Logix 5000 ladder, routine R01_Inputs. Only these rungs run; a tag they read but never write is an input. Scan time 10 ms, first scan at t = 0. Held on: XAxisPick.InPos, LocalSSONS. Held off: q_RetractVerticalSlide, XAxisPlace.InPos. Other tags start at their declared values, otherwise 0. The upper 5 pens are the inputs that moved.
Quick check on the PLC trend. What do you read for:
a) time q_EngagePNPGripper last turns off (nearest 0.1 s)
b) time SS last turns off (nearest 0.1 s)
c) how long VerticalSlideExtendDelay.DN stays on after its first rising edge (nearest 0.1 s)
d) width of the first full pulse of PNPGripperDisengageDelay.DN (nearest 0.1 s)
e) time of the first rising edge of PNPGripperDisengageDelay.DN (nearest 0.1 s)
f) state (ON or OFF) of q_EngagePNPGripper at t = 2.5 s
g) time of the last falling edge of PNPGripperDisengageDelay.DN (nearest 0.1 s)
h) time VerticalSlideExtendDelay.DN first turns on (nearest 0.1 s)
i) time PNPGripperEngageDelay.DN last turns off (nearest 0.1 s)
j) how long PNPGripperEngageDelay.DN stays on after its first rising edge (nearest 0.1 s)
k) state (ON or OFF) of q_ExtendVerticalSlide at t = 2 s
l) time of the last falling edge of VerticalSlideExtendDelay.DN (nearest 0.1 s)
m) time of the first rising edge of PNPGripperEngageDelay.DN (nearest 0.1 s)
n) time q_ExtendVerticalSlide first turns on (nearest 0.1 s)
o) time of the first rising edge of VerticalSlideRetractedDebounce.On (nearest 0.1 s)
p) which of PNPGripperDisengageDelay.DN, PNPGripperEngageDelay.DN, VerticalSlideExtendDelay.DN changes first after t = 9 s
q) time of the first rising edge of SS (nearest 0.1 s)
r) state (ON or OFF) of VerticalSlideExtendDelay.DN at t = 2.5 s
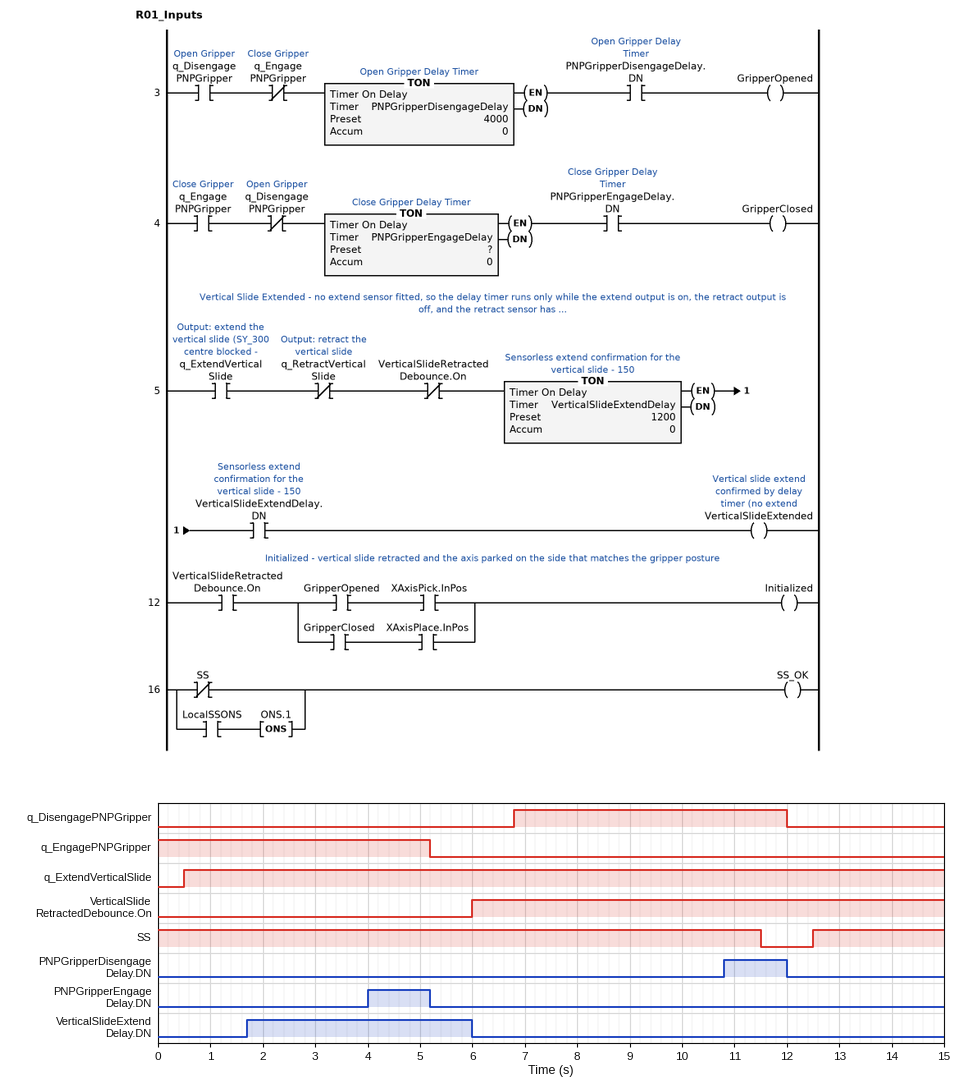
5.2 s
11.5 s
4.3 s
1.2 s
10.8 s
ON
12.0 s
1.7 s
5.2 s
1.2 s
ON
6.0 s
4.0 s
0.5 s
6.0 s
PNPGripperDisengageDelay.DN
12.5 s
ON
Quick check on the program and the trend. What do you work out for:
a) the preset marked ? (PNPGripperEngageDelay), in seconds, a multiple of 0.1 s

4.0 s
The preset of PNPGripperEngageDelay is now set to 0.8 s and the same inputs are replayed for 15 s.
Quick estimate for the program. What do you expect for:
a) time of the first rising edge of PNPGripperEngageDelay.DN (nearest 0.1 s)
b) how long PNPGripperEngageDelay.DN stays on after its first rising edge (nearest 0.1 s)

0.8 s
4.4 s
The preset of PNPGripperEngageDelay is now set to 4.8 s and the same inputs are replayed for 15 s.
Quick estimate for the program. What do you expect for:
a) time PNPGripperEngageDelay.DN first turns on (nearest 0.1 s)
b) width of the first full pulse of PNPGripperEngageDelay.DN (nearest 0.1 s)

4.8 s
0.4 s
